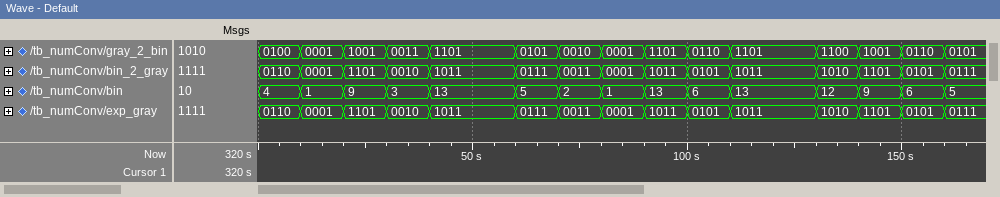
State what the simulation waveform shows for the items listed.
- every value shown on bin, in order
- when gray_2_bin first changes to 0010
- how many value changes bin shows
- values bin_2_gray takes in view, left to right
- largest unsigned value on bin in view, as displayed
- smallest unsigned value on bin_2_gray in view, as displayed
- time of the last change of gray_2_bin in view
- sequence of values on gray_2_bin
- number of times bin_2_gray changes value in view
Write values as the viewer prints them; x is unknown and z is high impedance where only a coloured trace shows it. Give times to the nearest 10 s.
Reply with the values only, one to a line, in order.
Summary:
4, 1, 9, 3, 13, 5, 2, 1, 13, 6, 13, 12, 9, 6, 5
70 s
14
0110, 0001, 1101, 0010, 1011, 0111, 0011, 0001, 1011, 0101, 1011, 1010, 1101, 0101, 0111
13
0001
160 s
0100, 0001, 1001, 0011, 1101, 0101, 0010, 0001, 1101, 0110, 1101, 1100, 1001, 0110, 0101
14
